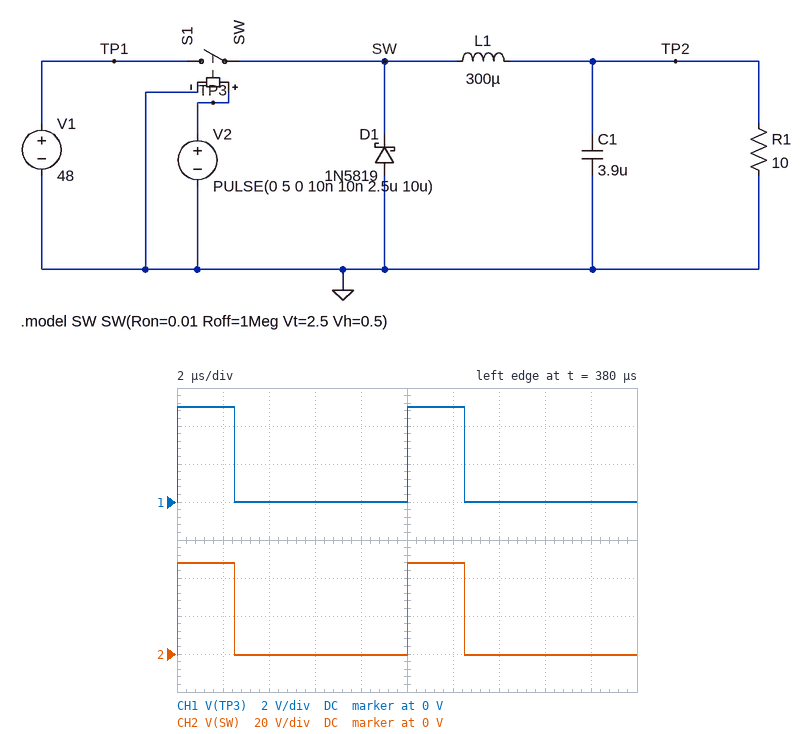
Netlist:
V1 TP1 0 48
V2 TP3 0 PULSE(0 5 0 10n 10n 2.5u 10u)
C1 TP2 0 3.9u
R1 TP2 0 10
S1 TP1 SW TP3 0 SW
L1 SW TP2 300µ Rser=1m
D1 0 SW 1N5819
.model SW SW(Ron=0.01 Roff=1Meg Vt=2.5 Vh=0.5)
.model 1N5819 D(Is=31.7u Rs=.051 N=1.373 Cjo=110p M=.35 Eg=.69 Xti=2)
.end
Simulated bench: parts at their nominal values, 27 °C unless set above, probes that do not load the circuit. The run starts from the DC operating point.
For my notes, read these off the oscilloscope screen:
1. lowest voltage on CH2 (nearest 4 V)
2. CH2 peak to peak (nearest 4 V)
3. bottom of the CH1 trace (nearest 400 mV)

0 V
48 V
0 V
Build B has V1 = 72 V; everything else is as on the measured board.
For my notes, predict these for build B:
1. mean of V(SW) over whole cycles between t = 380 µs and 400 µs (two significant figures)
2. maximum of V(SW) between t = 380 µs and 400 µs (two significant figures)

18 V
72 V
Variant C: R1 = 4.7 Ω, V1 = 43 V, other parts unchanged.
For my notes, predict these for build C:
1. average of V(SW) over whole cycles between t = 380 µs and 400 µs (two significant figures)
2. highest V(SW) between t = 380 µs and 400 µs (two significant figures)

10 V
43 V
